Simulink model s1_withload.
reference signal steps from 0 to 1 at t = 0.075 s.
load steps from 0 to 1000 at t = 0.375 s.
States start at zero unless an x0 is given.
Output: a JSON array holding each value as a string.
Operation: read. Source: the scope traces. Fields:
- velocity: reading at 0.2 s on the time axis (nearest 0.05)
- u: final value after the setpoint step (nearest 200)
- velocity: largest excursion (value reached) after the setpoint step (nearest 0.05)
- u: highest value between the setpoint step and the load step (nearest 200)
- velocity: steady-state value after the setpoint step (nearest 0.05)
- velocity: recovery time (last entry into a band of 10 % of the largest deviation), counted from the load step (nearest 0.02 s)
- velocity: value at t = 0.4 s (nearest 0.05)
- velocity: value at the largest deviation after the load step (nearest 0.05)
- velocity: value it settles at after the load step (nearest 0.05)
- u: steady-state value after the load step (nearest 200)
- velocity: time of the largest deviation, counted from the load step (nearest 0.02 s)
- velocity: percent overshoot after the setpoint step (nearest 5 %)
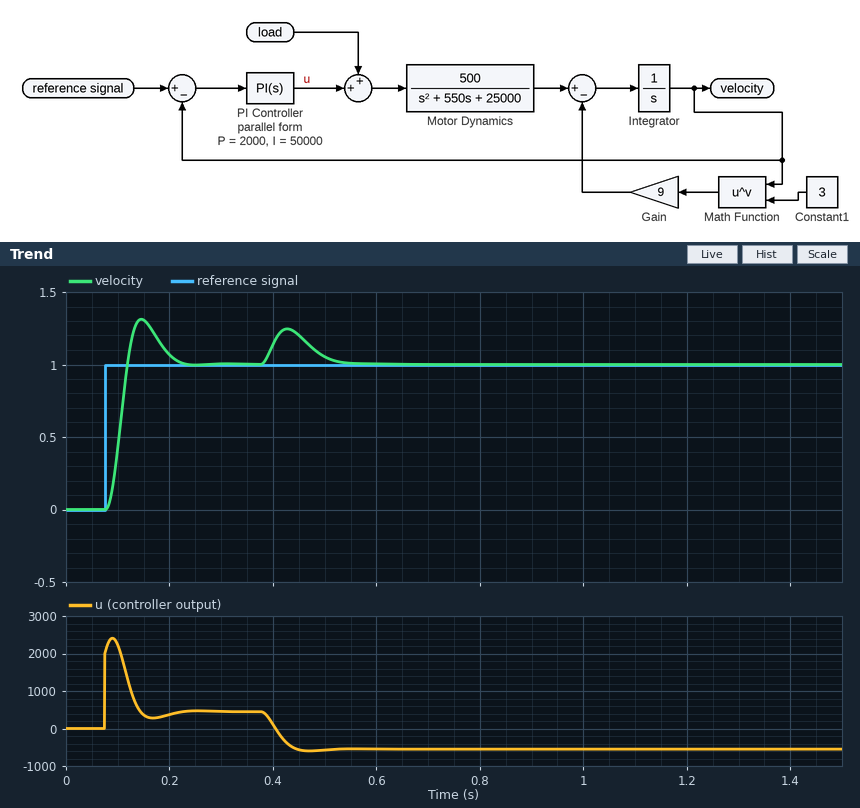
["1.05", "400", "1.30", "2400", "1.00", "0.14 s", "1.15", "1.25", "1.00", "-600", "0.06 s", "30 %"]
